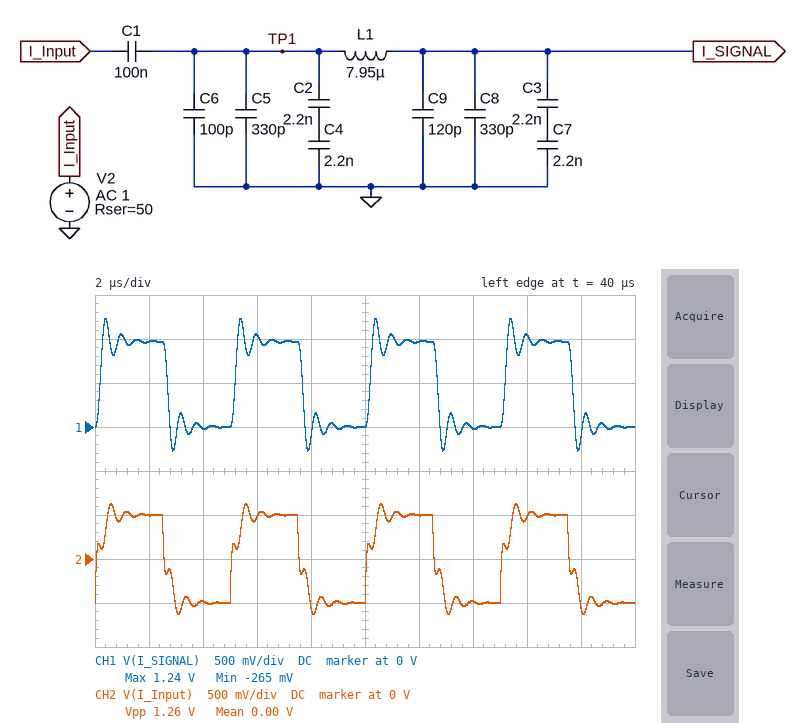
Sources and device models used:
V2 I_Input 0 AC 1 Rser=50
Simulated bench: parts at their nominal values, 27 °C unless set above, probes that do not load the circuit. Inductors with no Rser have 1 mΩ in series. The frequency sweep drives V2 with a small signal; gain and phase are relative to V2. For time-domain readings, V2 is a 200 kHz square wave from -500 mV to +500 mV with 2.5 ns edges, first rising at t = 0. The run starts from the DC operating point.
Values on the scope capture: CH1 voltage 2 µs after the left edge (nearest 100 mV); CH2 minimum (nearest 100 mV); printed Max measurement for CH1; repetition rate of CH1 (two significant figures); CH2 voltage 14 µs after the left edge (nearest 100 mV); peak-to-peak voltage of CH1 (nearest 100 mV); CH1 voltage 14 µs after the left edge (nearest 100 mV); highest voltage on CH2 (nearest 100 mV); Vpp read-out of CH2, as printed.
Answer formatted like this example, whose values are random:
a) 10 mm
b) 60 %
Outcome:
a) 1.0 V
b) -600 mV
c) 1.24 V
d) 200 kHz
e) -500 mV
f) 1.5 V
g) 0 V
h) 600 mV
i) 1.26 V
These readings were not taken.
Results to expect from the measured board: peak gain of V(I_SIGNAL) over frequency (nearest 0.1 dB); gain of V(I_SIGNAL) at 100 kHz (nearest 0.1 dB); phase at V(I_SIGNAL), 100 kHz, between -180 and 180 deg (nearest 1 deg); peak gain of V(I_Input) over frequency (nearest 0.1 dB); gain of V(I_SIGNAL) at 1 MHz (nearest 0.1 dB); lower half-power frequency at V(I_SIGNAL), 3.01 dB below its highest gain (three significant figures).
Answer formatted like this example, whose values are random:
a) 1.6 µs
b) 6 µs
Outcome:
a) 4.0 dB
b) -0.3 dB
c) -5 deg
d) 0 dB
e) 0.8 dB
f) 1.05 MHz
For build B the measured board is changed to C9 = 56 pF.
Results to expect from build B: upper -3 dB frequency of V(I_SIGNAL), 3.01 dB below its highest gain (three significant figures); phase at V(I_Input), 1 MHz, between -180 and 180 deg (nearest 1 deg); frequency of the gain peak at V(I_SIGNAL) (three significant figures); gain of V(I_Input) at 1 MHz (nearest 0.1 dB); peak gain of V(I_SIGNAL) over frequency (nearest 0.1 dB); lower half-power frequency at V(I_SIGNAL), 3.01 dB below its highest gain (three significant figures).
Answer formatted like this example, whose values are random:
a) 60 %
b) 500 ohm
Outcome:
a) 2.00 MHz
b) -52 deg
c) 1.69 MHz
d) -4.3 dB
e) 4.3 dB
f) 1.12 MHz
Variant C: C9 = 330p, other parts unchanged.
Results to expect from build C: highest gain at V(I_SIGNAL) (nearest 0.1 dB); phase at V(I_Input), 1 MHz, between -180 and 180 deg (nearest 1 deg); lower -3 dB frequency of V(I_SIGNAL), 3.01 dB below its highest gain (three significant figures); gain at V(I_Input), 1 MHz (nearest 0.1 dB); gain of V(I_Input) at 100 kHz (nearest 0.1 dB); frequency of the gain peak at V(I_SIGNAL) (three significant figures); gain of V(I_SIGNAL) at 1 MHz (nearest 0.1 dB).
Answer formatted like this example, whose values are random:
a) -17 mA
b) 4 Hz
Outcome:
a) 3.2 dB
b) -58 deg
c) 760 kHz
d) -5.6 dB
e) 0 dB
f) 1.55 MHz
g) 0.9 dB
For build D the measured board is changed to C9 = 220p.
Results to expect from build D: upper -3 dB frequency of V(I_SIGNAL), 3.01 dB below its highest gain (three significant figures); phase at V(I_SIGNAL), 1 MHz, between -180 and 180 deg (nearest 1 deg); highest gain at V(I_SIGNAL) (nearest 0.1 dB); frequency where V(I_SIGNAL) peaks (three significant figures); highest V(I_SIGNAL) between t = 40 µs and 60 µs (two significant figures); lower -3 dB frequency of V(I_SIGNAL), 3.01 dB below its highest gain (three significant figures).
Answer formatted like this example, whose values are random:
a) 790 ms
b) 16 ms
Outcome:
a) 1.93 MHz
b) -56 deg
c) 3.6 dB
d) 1.60 MHz
e) 1.2 V
f) 924 kHz
